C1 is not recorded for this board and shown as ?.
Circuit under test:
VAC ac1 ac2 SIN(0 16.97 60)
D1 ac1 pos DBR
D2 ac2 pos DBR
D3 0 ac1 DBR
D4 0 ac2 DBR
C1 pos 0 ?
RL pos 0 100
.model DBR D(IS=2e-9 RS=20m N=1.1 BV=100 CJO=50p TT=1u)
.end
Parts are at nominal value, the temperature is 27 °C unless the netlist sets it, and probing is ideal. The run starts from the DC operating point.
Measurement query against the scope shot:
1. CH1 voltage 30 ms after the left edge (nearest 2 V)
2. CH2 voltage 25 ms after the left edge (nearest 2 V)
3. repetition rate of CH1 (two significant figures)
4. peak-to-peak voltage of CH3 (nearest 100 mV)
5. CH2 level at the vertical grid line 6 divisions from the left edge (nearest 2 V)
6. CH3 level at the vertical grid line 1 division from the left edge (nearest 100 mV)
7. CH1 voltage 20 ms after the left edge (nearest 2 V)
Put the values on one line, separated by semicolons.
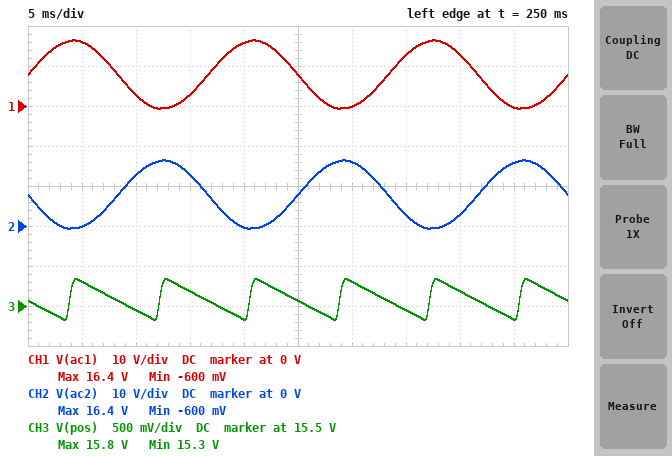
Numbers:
0 V; 8 V; 60 Hz; 500 mV; 16 V; 15.8 V; 16 V
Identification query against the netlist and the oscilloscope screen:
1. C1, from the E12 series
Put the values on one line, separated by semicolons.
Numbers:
2.2 mF
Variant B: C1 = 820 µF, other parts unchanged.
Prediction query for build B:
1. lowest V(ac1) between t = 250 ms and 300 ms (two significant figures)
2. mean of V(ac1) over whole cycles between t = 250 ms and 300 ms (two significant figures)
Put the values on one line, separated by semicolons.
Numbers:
-620 mV; 7.6 V
